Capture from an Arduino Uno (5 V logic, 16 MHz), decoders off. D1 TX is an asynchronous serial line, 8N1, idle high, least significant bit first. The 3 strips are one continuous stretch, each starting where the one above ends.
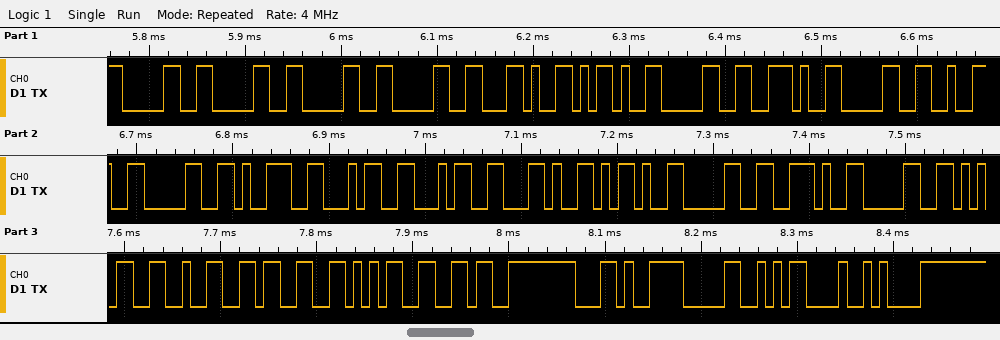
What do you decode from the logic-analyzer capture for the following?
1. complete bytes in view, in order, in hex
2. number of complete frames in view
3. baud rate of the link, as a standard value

0x30 0x30 0x30 0x30 0x2C 0x2D 0x30 0x2E 0x30 0x32 0x30 0x39 0x34 0x34 0x2C 0x2D 0x30 0x2E 0x30 0x35 0x32 0x33 0x35 0x36 0x2C 0x30 0x0D 0x0A
28
115200 baud
